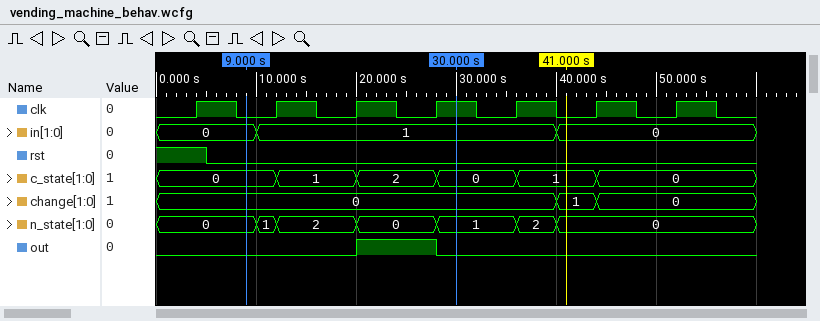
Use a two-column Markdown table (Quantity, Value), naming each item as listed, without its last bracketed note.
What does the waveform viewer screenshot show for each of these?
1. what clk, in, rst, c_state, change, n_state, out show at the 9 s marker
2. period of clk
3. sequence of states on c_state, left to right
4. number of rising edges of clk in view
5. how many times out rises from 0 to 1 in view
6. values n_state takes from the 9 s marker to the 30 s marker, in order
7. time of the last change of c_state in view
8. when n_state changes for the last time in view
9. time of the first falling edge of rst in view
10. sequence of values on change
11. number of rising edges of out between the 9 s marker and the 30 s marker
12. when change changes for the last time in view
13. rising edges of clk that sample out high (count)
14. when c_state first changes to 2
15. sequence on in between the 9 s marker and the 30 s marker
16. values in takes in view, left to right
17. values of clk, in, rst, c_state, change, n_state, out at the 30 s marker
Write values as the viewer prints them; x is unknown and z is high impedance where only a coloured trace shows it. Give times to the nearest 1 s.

| Quantity | Value |
|---|---|
| what clk, in, rst, c_state, change, n_state, out show at the 9 s marker | clk=0, in=0, rst=0, c_state=0, change=0, n_state=0, out=0 |
| period of clk | 8 s |
| sequence of states on c_state, left to right | 0, 1, 2, 0, 1, 0 |
| number of rising edges of clk in view | 7 |
| how many times out rises from 0 to 1 in view | 1 |
| values n_state takes from the 9 s marker to the 30 s marker, in order | 0, 1, 2, 0, 1 |
| time of the last change of c_state in view | 44 s |
| when n_state changes for the last time in view | 40 s |
| time of the first falling edge of rst in view | 5 s |
| sequence of values on change | 0, 1, 0 |
| number of rising edges of out between the 9 s marker and the 30 s marker | 1 |
| when change changes for the last time in view | 44 s |
| rising edges of clk that sample out high | 1 |
| when c_state first changes to 2 | 20 s |
| sequence on in between the 9 s marker and the 30 s marker | 0, 1 |
| values in takes in view, left to right | 0, 1, 0 |
| values of clk, in, rst, c_state, change, n_state, out at the 30 s marker | clk=1, in=1, rst=0, c_state=0, change=0, n_state=1, out=0 |
